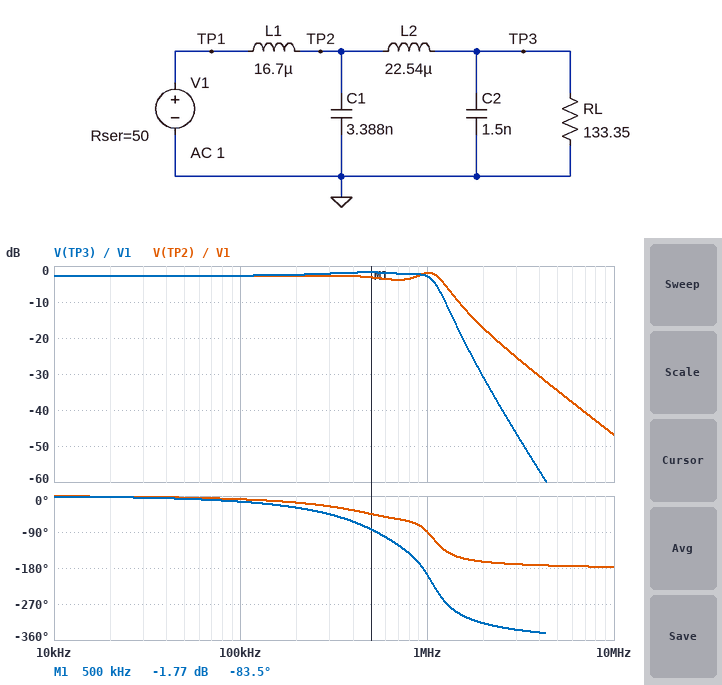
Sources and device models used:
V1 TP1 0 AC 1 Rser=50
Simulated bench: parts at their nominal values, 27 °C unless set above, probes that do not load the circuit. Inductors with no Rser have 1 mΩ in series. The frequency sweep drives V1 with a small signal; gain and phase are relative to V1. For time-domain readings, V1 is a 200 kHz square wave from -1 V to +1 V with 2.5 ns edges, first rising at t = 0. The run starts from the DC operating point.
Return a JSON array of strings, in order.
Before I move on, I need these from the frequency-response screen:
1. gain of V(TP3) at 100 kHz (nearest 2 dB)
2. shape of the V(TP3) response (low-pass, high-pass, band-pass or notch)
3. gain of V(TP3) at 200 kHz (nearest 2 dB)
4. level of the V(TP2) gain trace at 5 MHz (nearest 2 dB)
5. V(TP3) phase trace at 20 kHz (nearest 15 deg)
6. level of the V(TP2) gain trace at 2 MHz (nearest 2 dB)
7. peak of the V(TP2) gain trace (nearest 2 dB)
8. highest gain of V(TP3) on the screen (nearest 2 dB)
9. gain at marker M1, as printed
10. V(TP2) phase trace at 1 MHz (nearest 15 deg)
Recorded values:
["-2 dB", "low-pass", "-2 dB", "-34 dB", "0 deg", "-18 dB", "-2 dB", "-2 dB", "-1.77 dB", "-90 deg"]
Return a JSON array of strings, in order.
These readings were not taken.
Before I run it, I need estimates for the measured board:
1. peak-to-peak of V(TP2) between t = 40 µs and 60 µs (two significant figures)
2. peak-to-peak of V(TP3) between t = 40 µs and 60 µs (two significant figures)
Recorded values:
["1.7 V", "2.1 V"]
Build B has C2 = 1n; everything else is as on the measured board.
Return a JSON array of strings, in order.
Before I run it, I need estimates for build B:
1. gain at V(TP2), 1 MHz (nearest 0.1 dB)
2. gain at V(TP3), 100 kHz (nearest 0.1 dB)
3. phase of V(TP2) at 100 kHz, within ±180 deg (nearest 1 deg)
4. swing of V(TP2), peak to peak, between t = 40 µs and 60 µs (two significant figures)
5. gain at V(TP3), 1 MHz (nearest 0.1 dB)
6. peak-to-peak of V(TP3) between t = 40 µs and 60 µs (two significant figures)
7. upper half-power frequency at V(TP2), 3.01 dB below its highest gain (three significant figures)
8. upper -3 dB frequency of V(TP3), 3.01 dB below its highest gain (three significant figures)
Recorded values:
["-3.3 dB", "-2.7 dB", "-7 deg", "1.8 V", "-3.8 dB", "2.0 V", "1.19 MHz", "1.06 MHz"]
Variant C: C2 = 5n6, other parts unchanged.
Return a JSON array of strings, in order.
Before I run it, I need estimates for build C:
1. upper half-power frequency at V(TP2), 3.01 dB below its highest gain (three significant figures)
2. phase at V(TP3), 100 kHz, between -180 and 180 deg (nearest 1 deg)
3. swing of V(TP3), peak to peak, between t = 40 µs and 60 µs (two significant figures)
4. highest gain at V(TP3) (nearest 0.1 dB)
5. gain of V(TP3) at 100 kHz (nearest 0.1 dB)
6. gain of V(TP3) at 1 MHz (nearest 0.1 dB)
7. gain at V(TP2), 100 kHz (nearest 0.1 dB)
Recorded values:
["1.01 MHz", "-20 deg", "1.8 V", "-1.9 dB", "-2.5 dB", "-9.7 dB", "-2.9 dB"]
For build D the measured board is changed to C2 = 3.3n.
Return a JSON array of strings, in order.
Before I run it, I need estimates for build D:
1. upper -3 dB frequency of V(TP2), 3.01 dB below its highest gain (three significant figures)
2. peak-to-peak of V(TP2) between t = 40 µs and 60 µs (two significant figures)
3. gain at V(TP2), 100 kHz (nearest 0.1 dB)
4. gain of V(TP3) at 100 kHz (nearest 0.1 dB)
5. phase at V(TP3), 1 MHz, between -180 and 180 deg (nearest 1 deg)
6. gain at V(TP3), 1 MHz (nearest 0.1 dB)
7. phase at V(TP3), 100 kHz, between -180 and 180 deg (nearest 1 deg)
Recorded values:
["1.07 MHz", "2.1 V", "-2.8 dB", "-2.6 dB", "109 deg", "-4.3 dB", "-17 deg"]
